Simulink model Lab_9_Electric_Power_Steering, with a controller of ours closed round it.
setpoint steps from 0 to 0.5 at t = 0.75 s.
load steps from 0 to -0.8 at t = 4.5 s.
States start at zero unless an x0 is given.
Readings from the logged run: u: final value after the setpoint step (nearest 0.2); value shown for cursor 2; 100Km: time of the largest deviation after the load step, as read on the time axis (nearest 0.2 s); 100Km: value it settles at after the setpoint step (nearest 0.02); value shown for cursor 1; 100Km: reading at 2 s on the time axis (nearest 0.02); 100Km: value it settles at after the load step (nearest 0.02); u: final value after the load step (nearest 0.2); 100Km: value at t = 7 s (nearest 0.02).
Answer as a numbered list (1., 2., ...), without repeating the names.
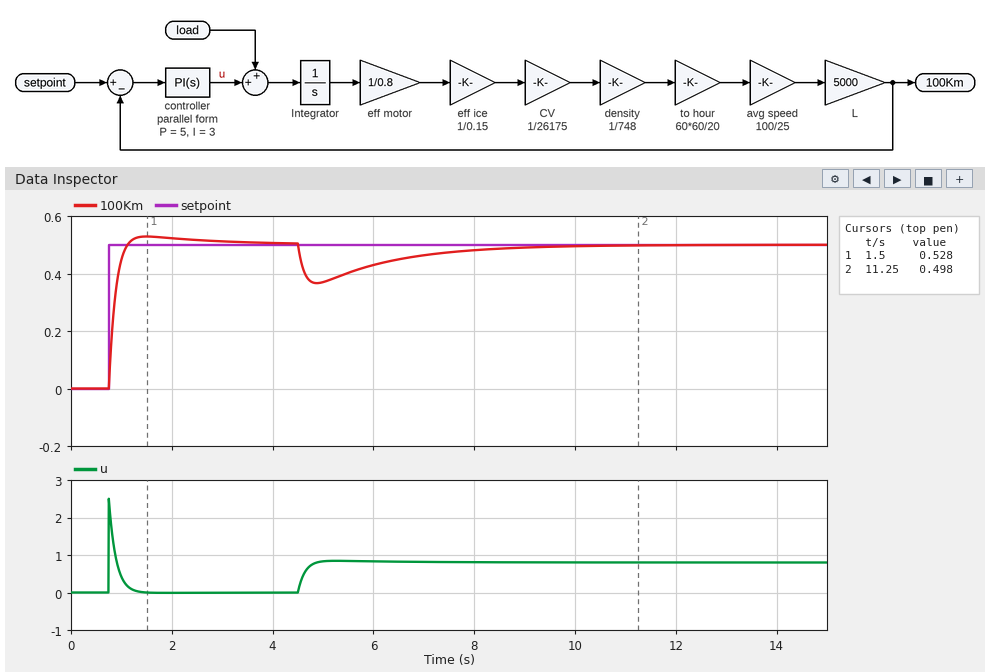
1. 0.0
2. 0.498
3. 4.8 s
4. 0.50
5. 0.528
6. 0.52
7. 0.50
8. 0.8
9. 0.46
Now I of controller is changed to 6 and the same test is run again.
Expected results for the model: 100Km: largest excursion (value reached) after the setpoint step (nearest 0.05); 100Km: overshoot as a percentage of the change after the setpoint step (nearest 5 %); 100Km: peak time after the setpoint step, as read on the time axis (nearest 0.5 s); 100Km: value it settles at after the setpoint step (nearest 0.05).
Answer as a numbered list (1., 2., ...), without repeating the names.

1. 0.55
2. 10 %
3. 1.5 s
4. 0.50
